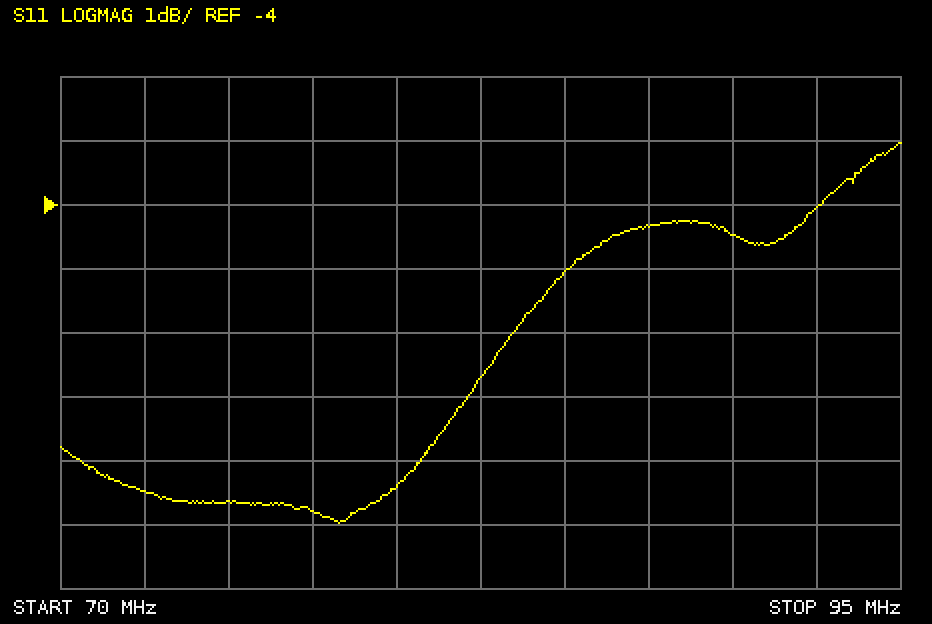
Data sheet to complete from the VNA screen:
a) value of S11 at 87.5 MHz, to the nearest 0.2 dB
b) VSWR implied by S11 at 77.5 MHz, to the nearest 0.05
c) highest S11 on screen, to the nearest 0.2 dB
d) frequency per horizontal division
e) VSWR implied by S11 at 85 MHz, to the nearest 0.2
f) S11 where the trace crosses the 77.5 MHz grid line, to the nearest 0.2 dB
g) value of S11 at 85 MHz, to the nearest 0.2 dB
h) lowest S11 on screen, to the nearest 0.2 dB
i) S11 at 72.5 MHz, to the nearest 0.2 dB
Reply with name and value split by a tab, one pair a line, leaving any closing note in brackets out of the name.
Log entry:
value of S11 at 87.5 MHz, to the nearest 0.2 dB	-4.4 dB
VSWR implied by S11 at 77.5 MHz, to the nearest 0.05	2.15
highest S11 on screen, to the nearest 0.2 dB	-3.0 dB
frequency per horizontal division	2.5 MHz
VSWR implied by S11 at 85 MHz, to the nearest 0.2	3.6
S11 where the trace crosses the 77.5 MHz grid line, to the nearest 0.2 dB	-8.8 dB
value of S11 at 85 MHz, to the nearest 0.2 dB	-5.0 dB
lowest S11 on screen, to the nearest 0.2 dB	-9.0 dB
S11 at 72.5 MHz, to the nearest 0.2 dB	-8.4 dB
